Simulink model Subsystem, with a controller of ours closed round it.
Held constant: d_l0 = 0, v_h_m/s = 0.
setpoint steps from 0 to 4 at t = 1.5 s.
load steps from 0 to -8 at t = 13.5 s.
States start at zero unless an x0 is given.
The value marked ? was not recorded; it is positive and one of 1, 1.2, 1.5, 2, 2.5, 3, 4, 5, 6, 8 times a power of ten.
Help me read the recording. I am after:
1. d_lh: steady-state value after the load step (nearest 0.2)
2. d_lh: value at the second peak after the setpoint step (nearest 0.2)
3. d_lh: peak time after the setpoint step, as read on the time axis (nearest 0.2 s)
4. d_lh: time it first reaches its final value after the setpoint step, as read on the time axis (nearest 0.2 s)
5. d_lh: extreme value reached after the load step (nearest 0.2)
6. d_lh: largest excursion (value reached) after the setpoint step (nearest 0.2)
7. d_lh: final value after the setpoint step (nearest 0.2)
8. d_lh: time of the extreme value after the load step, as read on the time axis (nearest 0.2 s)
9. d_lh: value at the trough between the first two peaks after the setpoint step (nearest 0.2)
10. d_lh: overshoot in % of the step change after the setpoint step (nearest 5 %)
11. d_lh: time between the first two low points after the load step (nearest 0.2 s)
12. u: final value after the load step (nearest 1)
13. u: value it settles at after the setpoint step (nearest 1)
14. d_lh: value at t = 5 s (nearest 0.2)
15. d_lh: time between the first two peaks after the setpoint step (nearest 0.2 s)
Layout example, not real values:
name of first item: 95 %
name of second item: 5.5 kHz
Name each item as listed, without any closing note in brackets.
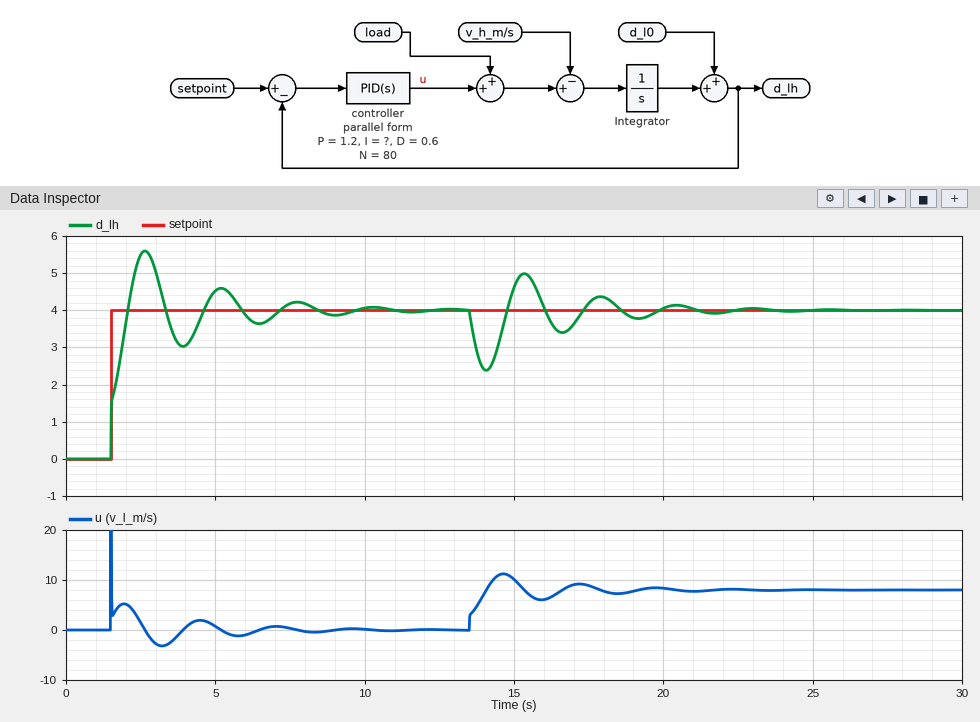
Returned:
d_lh: steady-state value after the load step: 4.0
d_lh: value at the second peak after the setpoint step: 4.6
d_lh: peak time after the setpoint step, as read on the time axis: 2.6 s
d_lh: time it first reaches its final value after the setpoint step, as read on the time axis: 2.0 s
d_lh: extreme value reached after the load step: 2.4
d_lh: largest excursion (value reached) after the setpoint step: 5.6
d_lh: final value after the setpoint step: 4.0
d_lh: time of the extreme value after the load step, as read on the time axis: 14.0 s
d_lh: value at the trough between the first two peaks after the setpoint step: 3.0
d_lh: overshoot in % of the step change after the setpoint step: 40 %
d_lh: time between the first two low points after the load step: 2.6 s
u: final value after the load step: 8
u: value it settles at after the setpoint step: 0
d_lh: value at t = 5 s: 4.6
d_lh: time between the first two peaks after the setpoint step: 2.6 s
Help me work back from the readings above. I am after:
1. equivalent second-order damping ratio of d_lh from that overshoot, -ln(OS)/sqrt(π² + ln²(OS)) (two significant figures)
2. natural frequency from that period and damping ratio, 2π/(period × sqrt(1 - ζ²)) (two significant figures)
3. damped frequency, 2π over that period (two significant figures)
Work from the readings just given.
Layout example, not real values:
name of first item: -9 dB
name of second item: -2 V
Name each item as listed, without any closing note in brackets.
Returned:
equivalent second-order damping ratio of d_lh from that overshoot, -ln(OS)/sqrt(π² + ln²(OS)): 0.28
natural frequency from that period and damping ratio, 2π/(period × sqrt(1 - ζ²)): 2.5 rad/s
damped frequency, 2π over that period: 2.4 rad/s
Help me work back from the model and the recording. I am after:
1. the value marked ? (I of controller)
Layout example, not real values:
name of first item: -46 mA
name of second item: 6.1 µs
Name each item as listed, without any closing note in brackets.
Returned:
the value marked ?: 10
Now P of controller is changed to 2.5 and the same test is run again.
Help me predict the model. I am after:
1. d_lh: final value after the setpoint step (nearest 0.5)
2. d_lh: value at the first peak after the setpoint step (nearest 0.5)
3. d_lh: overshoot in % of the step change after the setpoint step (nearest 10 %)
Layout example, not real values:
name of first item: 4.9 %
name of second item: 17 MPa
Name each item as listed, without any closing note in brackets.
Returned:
d_lh: final value after the setpoint step: 4.0
d_lh: value at the first peak after the setpoint step: 5.0
d_lh: overshoot in % of the step change after the setpoint step: 30 %
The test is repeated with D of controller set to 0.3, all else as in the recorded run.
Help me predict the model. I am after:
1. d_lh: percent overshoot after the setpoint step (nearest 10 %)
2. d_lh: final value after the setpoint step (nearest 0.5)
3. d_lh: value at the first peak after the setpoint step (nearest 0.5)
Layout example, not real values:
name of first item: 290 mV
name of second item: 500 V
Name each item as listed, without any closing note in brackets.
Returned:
d_lh: percent overshoot after the setpoint step: 50 %
d_lh: final value after the setpoint step: 4.0
d_lh: value at the first peak after the setpoint step: 6.0
